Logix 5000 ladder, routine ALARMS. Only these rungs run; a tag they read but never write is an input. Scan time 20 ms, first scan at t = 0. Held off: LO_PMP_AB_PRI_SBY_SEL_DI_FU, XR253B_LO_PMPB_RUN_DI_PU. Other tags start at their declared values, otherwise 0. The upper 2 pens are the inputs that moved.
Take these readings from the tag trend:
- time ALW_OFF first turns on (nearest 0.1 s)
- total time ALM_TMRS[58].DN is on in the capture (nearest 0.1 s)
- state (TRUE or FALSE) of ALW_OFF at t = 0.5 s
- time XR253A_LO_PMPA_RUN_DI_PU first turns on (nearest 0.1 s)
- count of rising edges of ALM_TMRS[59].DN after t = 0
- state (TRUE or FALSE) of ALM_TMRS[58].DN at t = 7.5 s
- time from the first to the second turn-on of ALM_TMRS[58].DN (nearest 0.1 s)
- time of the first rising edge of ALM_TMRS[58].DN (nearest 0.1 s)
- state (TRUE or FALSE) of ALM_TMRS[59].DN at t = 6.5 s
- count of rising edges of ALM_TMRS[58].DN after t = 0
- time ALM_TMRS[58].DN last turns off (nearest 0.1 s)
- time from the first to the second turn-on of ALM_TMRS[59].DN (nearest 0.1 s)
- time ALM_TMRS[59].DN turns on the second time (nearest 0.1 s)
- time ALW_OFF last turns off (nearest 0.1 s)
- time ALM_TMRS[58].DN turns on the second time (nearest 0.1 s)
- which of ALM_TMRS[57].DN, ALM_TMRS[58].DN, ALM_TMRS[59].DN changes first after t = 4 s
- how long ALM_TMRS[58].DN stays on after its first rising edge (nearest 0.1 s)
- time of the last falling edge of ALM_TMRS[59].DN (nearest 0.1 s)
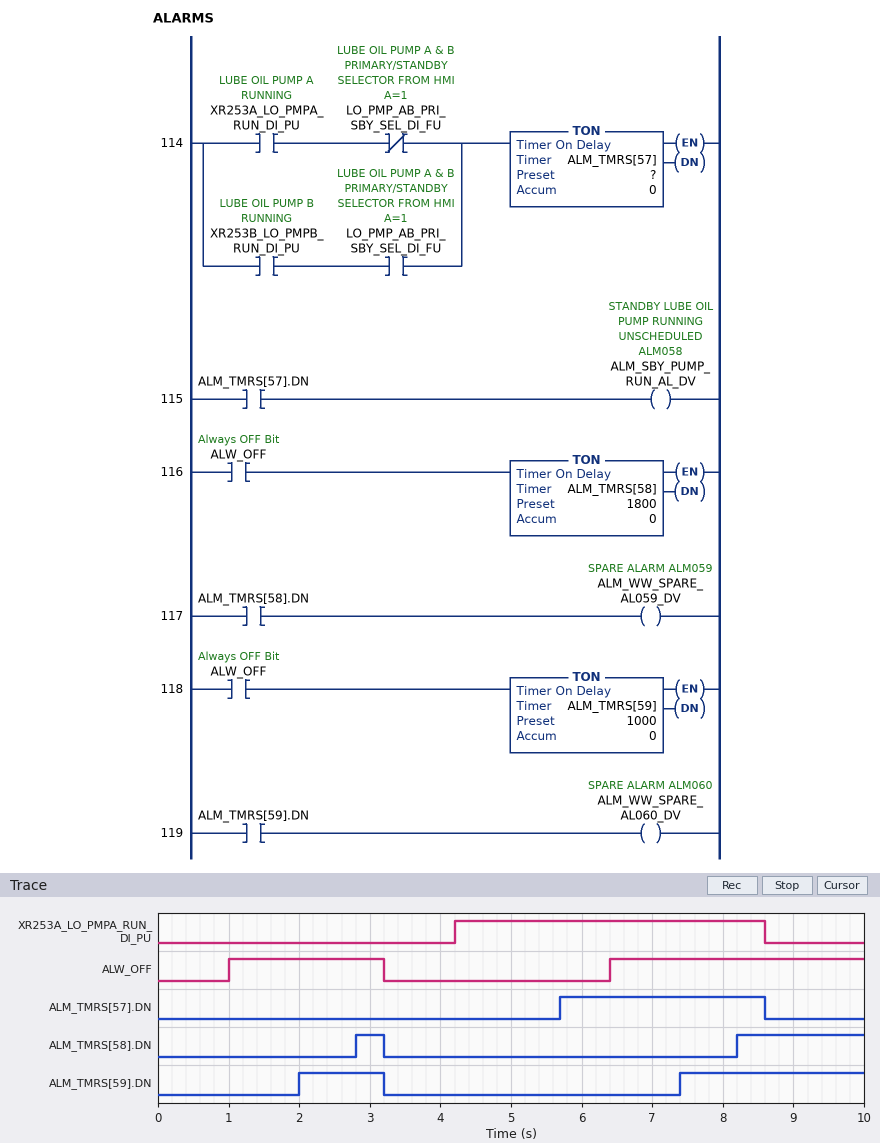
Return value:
1.0 s
2.2 s
FALSE
4.2 s
2
FALSE
5.4 s
2.8 s
FALSE
2
3.2 s
5.4 s
7.4 s
3.2 s
8.2 s
ALM_TMRS[57].DN
0.4 s
3.2 s
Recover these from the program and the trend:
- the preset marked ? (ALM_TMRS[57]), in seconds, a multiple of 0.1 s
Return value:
1.5 s
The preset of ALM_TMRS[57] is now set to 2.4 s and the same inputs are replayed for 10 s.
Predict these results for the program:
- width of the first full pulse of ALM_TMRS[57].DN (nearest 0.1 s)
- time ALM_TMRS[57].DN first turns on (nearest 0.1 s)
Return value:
2.0 s
6.6 s
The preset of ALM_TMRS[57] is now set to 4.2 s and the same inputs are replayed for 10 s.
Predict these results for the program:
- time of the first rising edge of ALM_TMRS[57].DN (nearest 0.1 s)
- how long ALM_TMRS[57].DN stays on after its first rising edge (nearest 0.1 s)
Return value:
8.4 s
0.2 s
